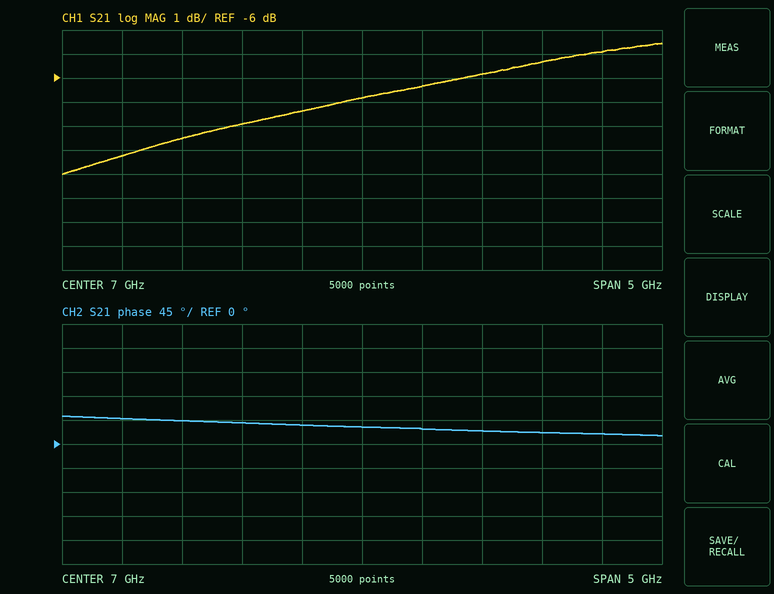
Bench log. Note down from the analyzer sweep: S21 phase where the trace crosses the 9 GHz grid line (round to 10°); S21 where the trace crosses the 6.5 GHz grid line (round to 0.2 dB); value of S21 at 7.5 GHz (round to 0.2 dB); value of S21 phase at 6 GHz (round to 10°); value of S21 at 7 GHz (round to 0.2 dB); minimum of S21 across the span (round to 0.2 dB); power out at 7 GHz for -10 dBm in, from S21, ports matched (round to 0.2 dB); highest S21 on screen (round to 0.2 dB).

20°
-7.4 dB
-6.4 dB
40°
-6.8 dB
-10.0 dB
-16.8 dBm
-4.6 dB
